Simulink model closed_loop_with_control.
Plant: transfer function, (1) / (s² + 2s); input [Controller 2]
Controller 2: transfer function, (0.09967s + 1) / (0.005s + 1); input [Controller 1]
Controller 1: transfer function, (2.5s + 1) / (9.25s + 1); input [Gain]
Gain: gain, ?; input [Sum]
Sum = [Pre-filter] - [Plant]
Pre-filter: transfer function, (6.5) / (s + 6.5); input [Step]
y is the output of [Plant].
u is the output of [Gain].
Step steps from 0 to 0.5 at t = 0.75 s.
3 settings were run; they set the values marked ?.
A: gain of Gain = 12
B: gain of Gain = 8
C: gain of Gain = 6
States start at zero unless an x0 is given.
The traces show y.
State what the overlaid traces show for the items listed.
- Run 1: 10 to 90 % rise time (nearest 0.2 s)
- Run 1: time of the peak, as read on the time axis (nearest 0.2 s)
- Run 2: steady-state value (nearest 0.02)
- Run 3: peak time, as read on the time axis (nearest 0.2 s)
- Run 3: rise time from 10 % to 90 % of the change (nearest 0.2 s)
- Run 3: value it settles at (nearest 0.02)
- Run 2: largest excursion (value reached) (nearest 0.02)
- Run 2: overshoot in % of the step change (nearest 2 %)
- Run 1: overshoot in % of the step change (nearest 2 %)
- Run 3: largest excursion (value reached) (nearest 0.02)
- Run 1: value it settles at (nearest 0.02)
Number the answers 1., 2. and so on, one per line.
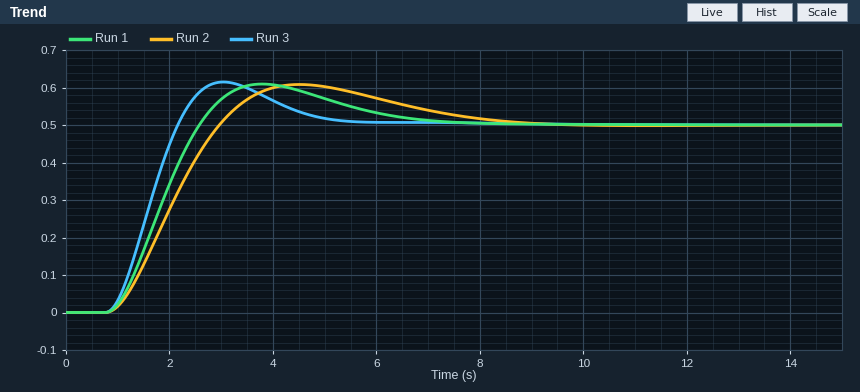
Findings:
1. 1.2 s
2. 3.8 s
3. 0.50
4. 3.0 s
5. 1.0 s
6. 0.50
7. 0.60
8. 22 %
9. 22 %
10. 0.62
11. 0.50
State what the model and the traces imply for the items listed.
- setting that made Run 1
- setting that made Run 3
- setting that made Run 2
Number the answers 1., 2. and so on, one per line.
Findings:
1. B
2. A
3. C
